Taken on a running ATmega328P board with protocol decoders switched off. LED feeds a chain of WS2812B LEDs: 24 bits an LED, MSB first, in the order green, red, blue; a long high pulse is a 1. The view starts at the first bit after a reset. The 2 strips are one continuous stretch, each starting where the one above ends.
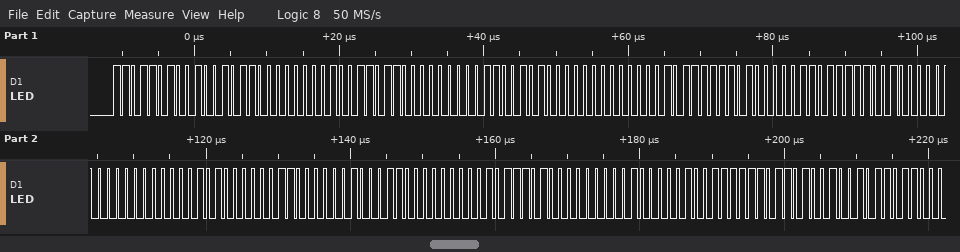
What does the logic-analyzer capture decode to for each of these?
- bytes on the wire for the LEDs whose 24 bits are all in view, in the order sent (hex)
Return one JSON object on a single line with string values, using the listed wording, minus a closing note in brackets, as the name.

{"bytes on the wire for the LEDs whose 24 bits are all in view, in the order sent": "DA 4B 00 9B 00 65 00 05 FA 0D F2 00 00 A0 60 46 00 BA 00 82 7E"}
